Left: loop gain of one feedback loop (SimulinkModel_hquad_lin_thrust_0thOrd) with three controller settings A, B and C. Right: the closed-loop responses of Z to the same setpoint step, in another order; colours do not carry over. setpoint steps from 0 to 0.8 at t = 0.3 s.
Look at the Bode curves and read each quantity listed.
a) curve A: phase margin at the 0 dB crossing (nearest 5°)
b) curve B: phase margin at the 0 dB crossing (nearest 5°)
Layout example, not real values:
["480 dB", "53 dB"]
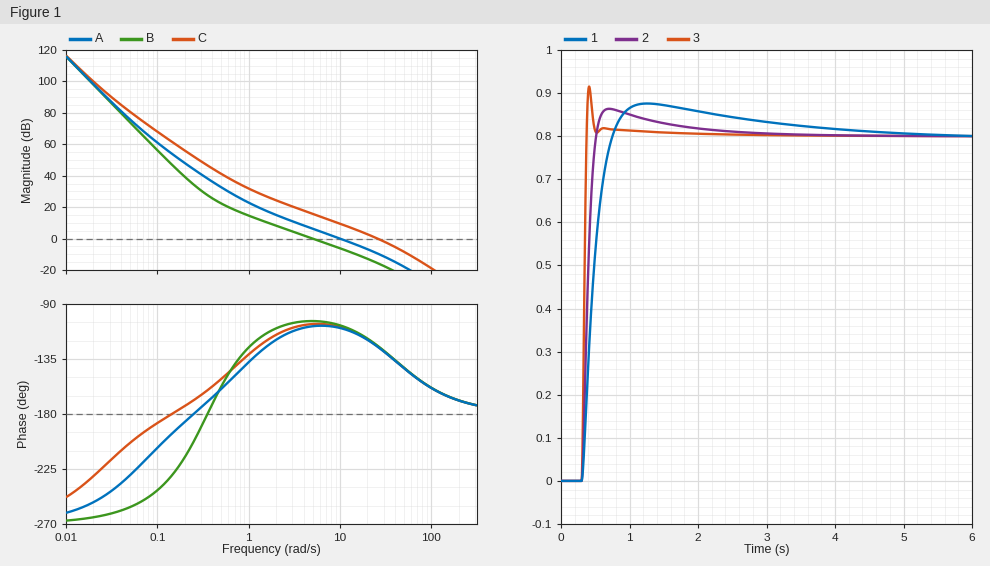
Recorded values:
["70°", "75°"]
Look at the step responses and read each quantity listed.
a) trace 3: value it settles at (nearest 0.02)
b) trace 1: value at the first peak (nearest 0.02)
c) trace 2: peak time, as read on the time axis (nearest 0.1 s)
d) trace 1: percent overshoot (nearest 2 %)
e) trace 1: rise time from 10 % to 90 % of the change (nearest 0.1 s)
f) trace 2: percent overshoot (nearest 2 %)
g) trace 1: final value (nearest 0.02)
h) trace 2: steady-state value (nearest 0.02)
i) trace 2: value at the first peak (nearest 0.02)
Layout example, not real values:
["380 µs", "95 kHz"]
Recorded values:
["0.80", "0.88", "0.7 s", "10 %", "0.3 s", "8 %", "0.80", "0.80", "0.86"]
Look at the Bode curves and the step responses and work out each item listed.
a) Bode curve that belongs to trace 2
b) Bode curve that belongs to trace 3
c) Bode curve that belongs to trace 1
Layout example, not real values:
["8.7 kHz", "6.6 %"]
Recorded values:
["A", "C", "B"]
